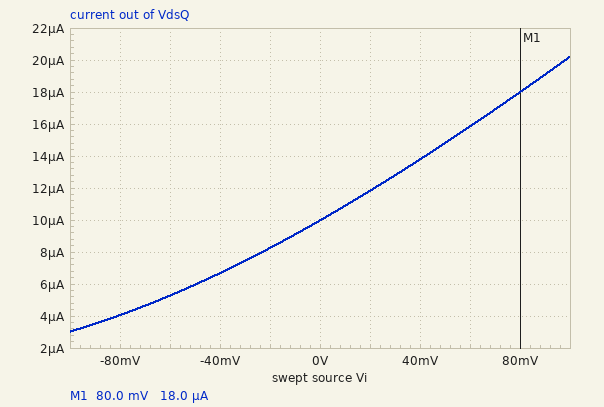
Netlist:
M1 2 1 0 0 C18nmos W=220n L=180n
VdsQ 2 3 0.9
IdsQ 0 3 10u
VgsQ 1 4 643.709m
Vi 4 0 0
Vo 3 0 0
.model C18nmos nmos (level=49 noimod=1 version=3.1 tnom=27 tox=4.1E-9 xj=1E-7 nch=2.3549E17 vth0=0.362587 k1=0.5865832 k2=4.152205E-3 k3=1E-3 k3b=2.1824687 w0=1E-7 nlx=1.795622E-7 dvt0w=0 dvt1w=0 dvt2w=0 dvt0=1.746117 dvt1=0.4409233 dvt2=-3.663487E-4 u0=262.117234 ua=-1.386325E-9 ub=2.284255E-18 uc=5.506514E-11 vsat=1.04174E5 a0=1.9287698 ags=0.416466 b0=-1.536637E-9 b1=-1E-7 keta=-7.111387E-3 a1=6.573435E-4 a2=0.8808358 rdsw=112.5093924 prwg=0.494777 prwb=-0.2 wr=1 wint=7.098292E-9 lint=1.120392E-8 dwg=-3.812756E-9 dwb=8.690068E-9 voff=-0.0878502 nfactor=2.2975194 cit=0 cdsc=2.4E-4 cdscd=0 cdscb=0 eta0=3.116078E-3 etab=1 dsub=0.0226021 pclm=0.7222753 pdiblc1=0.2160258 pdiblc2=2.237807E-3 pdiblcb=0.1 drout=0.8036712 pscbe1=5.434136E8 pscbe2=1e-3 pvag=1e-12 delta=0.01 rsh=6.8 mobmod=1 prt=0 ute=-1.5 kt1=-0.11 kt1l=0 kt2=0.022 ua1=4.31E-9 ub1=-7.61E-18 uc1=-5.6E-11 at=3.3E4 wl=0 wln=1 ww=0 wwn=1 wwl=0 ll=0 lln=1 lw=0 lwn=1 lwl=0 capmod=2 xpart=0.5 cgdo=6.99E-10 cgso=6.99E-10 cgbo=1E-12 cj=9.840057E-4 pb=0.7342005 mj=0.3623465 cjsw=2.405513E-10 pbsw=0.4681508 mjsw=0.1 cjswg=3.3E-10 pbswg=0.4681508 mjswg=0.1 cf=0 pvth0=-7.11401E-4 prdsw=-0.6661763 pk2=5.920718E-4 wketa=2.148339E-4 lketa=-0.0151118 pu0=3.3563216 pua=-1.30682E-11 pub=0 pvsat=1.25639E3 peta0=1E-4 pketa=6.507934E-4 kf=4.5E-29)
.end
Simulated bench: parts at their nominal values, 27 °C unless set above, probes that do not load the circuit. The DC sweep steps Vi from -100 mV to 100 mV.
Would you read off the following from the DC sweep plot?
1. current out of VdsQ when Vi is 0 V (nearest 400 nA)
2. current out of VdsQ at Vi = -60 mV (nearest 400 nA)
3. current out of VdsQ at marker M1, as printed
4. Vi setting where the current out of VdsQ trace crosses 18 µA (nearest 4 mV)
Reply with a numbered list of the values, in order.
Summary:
1. 10.0 µA
2. 5.2 µA
3. 18.0 µA
4. 80 mV
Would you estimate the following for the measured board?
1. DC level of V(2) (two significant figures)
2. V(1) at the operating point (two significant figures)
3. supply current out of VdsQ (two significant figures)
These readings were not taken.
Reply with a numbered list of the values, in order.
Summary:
1. 900 mV
2. 640 mV
3. 10 µA
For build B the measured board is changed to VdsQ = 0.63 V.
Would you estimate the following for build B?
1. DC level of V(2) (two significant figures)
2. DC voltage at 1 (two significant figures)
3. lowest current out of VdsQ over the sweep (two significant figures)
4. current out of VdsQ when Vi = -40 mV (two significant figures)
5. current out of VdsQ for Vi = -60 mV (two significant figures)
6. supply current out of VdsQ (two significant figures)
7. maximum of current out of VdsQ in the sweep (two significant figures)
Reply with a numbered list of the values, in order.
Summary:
1. 630 mV
2. 640 mV
3. 2.6 µA
4. 6.0 µA
5. 4.7 µA
6. 9.1 µA
7. 19 µA
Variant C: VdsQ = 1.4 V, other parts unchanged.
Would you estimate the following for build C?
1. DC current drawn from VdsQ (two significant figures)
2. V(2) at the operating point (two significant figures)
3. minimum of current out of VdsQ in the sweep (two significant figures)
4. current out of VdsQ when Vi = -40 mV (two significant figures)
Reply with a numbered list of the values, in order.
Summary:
1. 12 µA
2. 1.4 V
3. 3.9 µA
4. 8.0 µA
